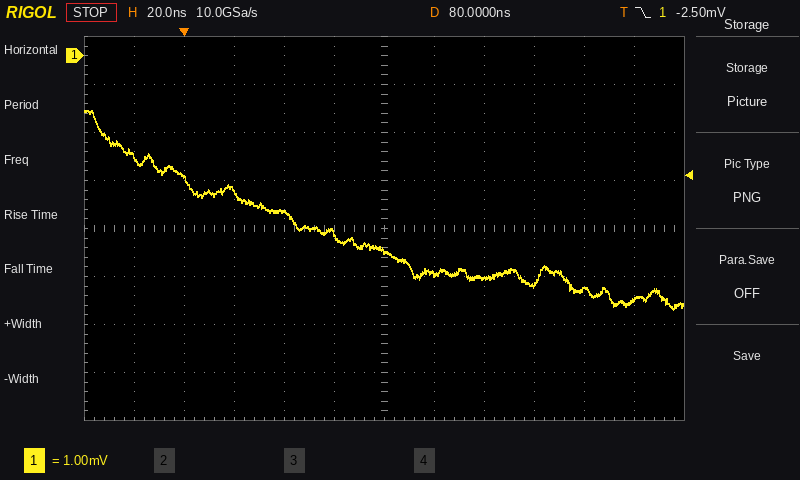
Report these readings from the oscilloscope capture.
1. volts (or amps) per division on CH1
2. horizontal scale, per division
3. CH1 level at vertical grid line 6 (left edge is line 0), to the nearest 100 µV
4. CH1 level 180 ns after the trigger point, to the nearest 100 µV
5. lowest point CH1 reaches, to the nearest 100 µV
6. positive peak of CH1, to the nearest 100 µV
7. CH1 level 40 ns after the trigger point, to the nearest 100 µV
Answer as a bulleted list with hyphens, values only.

- 1 mV
- 20 ns
- -4.1 mV
- -5.1 mV
- -5.3 mV
- -1.1 mV
- -3.3 mV
